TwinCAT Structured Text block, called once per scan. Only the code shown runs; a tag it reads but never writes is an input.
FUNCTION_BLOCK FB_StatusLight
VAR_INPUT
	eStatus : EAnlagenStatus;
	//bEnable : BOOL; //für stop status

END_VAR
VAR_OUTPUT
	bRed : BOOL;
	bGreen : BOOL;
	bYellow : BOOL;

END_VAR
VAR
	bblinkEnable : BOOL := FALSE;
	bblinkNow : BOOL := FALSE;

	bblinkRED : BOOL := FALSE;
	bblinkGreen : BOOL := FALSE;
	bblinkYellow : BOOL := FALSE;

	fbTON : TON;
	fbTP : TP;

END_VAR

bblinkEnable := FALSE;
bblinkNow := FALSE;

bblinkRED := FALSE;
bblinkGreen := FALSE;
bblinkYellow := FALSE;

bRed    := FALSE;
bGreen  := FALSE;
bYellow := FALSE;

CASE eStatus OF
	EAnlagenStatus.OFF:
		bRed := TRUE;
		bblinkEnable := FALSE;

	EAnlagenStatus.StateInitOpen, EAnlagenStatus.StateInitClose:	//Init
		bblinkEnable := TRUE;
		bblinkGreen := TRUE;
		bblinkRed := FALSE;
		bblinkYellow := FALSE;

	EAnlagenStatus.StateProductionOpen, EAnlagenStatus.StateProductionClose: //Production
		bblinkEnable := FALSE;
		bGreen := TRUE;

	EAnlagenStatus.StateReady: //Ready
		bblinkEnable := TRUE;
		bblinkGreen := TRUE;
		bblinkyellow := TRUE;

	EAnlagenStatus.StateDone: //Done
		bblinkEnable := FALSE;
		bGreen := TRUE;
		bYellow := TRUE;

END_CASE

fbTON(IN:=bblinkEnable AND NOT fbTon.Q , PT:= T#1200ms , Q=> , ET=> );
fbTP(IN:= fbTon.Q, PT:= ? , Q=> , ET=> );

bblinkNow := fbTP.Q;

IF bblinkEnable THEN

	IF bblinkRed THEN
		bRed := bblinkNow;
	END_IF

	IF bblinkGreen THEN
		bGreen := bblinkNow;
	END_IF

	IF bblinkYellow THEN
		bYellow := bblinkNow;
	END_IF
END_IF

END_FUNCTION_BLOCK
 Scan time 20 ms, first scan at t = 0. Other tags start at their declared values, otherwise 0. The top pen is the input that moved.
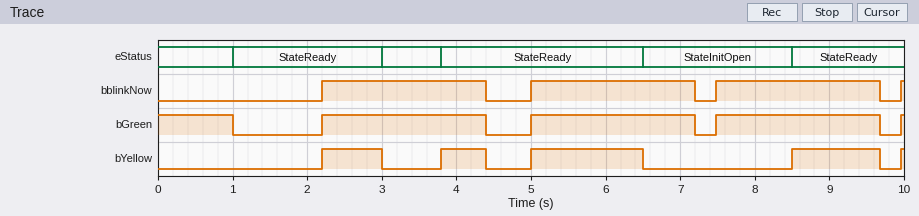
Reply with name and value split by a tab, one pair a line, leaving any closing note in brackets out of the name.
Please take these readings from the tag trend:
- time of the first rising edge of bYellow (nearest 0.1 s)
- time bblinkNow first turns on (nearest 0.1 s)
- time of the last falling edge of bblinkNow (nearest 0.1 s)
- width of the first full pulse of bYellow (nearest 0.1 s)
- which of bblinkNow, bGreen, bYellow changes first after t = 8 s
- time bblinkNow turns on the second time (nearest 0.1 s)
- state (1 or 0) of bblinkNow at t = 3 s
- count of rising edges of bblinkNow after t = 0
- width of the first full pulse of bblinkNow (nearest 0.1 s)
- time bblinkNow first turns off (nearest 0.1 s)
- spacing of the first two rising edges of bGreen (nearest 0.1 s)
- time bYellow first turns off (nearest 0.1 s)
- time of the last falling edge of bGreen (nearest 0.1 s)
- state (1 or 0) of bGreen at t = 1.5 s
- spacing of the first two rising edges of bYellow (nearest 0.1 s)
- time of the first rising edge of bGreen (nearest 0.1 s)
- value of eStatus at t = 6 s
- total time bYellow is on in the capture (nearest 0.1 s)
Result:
time of the first rising edge of bYellow	2.2 s
time bblinkNow first turns on	2.2 s
time of the last falling edge of bblinkNow	9.7 s
width of the first full pulse of bYellow	0.8 s
which of bblinkNow, bGreen, bYellow changes first after t = 8 s	bYellow
time bblinkNow turns on the second time	5.0 s
state (1 or 0) of bblinkNow at t = 3 s	1
count of rising edges of bblinkNow after t = 0	4
width of the first full pulse of bblinkNow	2.2 s
time bblinkNow first turns off	4.4 s
spacing of the first two rising edges of bGreen	2.8 s
time bYellow first turns off	3.0 s
time of the last falling edge of bGreen	9.7 s
state (1 or 0) of bGreen at t = 1.5 s	0
spacing of the first two rising edges of bYellow	1.6 s
time of the first rising edge of bGreen	2.2 s
value of eStatus at t = 6 s	StateReady
total time bYellow is on in the capture	4.1 s
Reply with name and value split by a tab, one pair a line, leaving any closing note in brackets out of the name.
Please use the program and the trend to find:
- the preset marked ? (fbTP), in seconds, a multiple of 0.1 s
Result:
the preset marked ? (fbTP), in seconds, a multiple of 0.1 s	2.2 s
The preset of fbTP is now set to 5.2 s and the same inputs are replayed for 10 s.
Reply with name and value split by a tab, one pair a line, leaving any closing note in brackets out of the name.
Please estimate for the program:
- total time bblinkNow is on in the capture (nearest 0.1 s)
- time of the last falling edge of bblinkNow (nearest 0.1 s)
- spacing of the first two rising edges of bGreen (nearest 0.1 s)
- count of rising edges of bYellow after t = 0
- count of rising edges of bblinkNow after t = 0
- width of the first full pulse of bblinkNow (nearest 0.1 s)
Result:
total time bblinkNow is on in the capture	7.7 s
time of the last falling edge of bblinkNow	7.4 s
spacing of the first two rising edges of bGreen	5.3 s
count of rising edges of bYellow after t = 0	3
count of rising edges of bblinkNow after t = 0	2
width of the first full pulse of bblinkNow	5.2 s
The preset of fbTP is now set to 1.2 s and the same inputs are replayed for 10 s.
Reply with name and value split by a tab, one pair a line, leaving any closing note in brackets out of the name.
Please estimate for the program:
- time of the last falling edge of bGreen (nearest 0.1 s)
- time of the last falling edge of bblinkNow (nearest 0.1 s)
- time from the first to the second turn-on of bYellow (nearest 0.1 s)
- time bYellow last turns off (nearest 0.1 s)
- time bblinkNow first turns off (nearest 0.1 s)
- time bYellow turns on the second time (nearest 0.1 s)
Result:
time of the last falling edge of bGreen	9.9 s
time of the last falling edge of bblinkNow	9.9 s
time from the first to the second turn-on of bYellow	2.8 s
time bYellow last turns off	9.9 s
time bblinkNow first turns off	3.4 s
time bYellow turns on the second time	5.0 s
